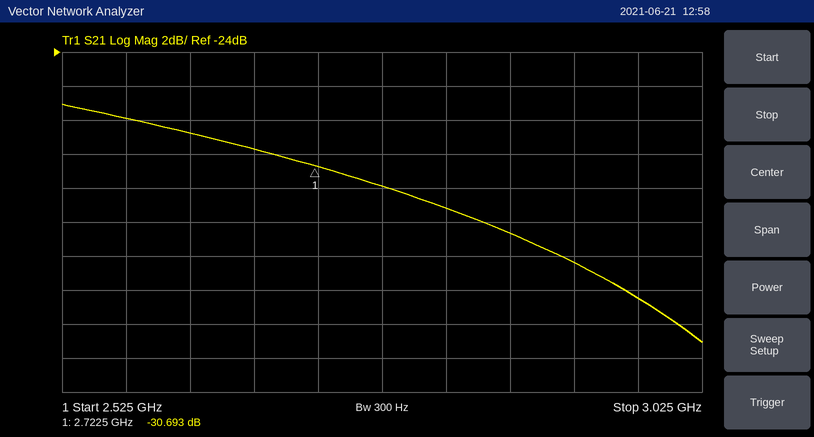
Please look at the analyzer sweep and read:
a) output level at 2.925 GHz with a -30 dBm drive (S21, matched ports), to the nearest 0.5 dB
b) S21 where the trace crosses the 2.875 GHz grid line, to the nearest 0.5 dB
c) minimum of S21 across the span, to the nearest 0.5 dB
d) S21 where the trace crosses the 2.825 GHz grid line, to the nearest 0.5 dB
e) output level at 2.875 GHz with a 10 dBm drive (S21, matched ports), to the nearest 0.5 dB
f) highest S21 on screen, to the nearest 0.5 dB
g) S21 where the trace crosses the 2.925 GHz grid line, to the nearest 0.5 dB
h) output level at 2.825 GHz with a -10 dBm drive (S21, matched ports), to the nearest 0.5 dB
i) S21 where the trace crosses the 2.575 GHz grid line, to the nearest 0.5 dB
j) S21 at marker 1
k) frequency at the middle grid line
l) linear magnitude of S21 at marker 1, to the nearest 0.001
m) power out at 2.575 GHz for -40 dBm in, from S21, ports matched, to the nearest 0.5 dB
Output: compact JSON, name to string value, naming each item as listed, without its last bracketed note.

{"output level at 2.925 GHz with a -30 dBm drive (S21, matched ports), to the nearest 0.5 dB": "-66.5 dBm", "S21 where the trace crosses the 2.875 GHz grid line, to the nearest 0.5 dB": "-34.5 dB", "minimum of S21 across the span, to the nearest 0.5 dB": "-41.0 dB", "S21 where the trace crosses the 2.825 GHz grid line, to the nearest 0.5 dB": "-33.0 dB", "output level at 2.875 GHz with a 10 dBm drive (S21, matched ports), to the nearest 0.5 dB": "-24.5 dBm", "highest S21 on screen, to the nearest 0.5 dB": "-27.0 dB", "S21 where the trace crosses the 2.925 GHz grid line, to the nearest 0.5 dB": "-36.5 dB", "output level at 2.825 GHz with a -10 dBm drive (S21, matched ports), to the nearest 0.5 dB": "-43.0 dBm", "S21 where the trace crosses the 2.575 GHz grid line, to the nearest 0.5 dB": "-28.0 dB", "S21 at marker 1": "-30.693 dB", "frequency at the middle grid line": "2.775 GHz", "linear magnitude of S21 at marker 1, to the nearest 0.001": "0.029", "power out at 2.575 GHz for -40 dBm in, from S21, ports matched, to the nearest 0.5 dB": "-68.0 dBm"}
